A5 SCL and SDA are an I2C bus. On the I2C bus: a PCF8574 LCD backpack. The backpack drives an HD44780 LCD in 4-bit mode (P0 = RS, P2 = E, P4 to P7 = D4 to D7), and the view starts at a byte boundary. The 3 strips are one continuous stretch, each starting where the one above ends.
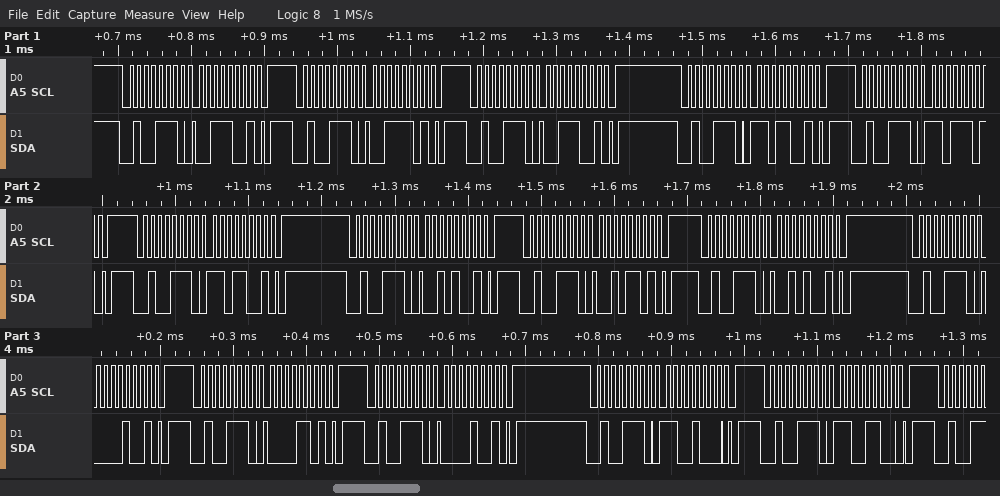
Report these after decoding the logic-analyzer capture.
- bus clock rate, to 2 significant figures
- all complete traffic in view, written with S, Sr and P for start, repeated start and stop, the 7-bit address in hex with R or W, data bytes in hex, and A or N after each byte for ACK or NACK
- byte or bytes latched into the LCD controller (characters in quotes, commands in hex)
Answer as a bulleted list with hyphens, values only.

- 100 kHz
- S 27W A 39 A P S 27W A 3D A P S 27W A 39 A P S 27W A D9 A P S 27W A DD A P S 27W A D9 A P S 27W A 29 A P S 27W A 2D A P S 27W A 29 A P S 27W A 09 A P S 27W A 0D A P S 27W A 09 A P S 27W A C8 A P S 27W A CC A P
- '=' ' '
